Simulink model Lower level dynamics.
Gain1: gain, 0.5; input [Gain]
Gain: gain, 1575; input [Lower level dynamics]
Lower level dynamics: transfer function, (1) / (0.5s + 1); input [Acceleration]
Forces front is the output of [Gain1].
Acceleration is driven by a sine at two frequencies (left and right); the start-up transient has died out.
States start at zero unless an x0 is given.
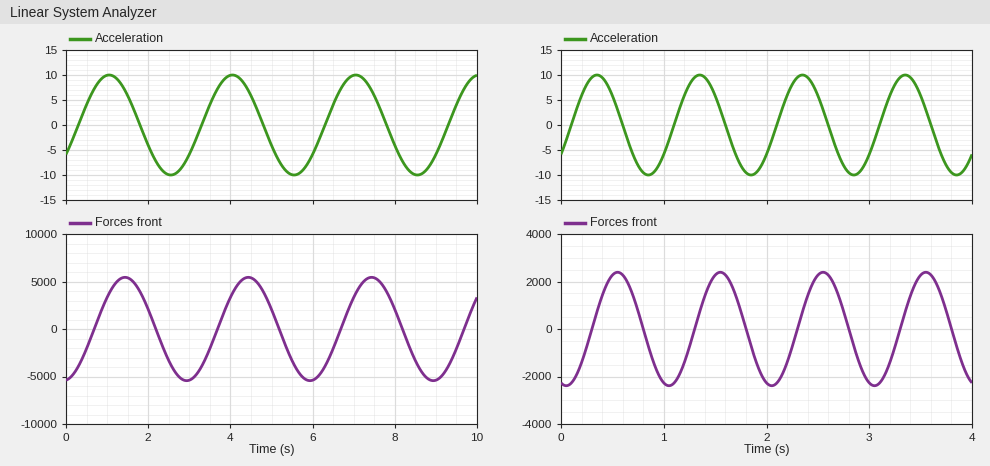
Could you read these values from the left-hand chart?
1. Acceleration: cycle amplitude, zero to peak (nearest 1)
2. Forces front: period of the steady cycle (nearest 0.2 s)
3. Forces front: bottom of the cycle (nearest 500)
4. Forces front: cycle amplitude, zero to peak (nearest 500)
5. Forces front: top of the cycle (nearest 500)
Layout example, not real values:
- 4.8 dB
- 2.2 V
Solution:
- 10
- 3.0 s
- -5500
- 5500
- 5500
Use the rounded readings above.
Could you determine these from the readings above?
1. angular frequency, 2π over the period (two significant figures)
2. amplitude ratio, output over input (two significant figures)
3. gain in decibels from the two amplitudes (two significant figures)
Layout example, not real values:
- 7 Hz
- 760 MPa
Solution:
- 2.1 rad/s
- 550
- 55 dB
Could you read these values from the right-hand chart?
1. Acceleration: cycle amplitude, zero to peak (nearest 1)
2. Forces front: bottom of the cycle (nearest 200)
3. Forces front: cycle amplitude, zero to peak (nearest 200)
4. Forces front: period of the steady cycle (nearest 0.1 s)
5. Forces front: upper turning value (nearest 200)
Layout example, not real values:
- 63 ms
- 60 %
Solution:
- 10
- -2400
- 2400
- 1.0 s
- 2400
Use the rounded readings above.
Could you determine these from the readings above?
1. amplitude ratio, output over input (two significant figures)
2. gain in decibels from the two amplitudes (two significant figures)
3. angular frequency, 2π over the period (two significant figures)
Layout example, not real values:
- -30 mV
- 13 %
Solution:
- 240
- 48 dB
- 6.3 rad/s
